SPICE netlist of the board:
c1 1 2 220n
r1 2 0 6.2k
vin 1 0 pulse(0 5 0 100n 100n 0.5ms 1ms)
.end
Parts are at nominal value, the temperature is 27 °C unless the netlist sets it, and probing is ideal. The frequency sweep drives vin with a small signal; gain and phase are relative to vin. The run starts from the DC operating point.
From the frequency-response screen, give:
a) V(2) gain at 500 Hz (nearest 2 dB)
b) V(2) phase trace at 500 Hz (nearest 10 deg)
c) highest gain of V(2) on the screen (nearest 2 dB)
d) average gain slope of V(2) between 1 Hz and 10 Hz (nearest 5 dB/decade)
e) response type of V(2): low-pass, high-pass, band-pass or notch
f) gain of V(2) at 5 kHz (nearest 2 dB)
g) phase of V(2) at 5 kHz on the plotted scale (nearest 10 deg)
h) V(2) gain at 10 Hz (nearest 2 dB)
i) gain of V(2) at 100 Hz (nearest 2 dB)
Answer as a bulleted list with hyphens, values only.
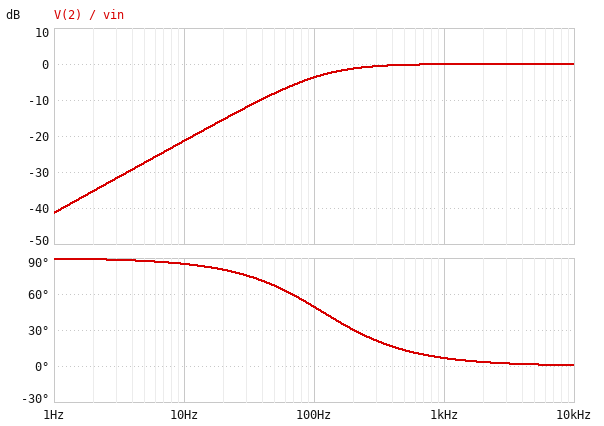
- 0 dB
- 10 deg
- 0 dB
- 20 dB/decade
- high-pass
- 0 dB
- 0 deg
- -22 dB
- -4 dB
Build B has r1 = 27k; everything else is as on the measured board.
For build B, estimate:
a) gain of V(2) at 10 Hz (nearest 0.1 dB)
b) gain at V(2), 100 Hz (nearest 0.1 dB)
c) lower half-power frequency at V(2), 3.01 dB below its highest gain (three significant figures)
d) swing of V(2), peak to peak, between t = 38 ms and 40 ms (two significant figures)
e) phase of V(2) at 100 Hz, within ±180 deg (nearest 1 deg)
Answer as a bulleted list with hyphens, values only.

- -9.1 dB
- -0.3 dB
- 26.8 Hz
- 5.2 V
- 15 deg
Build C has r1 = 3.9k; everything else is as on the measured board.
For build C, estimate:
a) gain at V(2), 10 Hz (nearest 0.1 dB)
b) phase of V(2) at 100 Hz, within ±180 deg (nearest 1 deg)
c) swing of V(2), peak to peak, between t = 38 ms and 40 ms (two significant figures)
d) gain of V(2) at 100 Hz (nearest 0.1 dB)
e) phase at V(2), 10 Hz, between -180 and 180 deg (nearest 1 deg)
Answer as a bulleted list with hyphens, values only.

- -25.4 dB
- 62 deg
- 6.4 V
- -6.5 dB
- 87 deg
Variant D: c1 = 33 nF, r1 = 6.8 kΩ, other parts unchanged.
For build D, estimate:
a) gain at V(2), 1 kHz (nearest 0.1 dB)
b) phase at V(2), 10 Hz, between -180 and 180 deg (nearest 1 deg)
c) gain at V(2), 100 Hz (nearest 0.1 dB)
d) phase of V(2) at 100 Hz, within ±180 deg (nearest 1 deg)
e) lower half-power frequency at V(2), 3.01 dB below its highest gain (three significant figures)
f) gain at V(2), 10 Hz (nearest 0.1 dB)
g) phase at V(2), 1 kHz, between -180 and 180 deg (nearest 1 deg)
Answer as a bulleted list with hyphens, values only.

- -1.8 dB
- 89 deg
- -17.1 dB
- 82 deg
- 709 Hz
- -37.0 dB
- 35 deg
